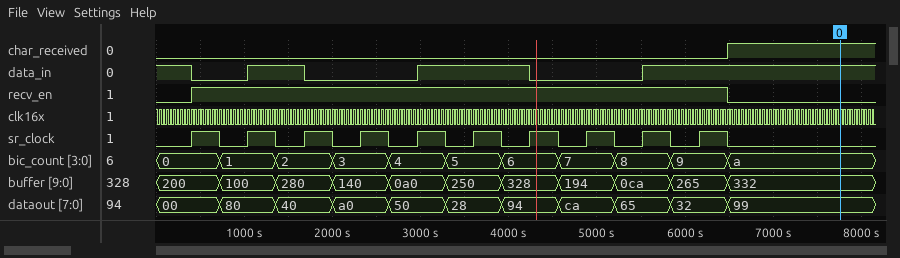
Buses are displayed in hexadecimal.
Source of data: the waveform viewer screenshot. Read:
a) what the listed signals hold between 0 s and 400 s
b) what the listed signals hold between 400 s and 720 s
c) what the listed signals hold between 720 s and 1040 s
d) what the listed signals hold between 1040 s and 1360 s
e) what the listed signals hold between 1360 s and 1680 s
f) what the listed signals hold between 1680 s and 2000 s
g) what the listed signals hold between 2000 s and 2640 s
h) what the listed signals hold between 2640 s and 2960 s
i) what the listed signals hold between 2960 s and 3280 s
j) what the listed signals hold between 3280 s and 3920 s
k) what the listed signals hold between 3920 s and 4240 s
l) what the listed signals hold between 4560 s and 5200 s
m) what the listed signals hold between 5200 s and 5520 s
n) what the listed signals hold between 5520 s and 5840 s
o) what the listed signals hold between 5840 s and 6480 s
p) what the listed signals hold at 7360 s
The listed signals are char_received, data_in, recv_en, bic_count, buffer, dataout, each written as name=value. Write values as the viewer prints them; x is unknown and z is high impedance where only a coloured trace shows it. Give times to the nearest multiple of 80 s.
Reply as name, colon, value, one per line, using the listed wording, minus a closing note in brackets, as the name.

what the listed signals hold between 0 s and 400 s: char_received=0, data_in=1, recv_en=0, bic_count=0, buffer=200, dataout=00
what the listed signals hold between 400 s and 720 s: char_received=0, data_in=0, recv_en=1, bic_count=0, buffer=200, dataout=00
what the listed signals hold between 720 s and 1040 s: char_received=0, data_in=0, recv_en=1, bic_count=1, buffer=100, dataout=80
what the listed signals hold between 1040 s and 1360 s: char_received=0, data_in=1, recv_en=1, bic_count=1, buffer=100, dataout=80
what the listed signals hold between 1360 s and 1680 s: char_received=0, data_in=1, recv_en=1, bic_count=2, buffer=280, dataout=40
what the listed signals hold between 1680 s and 2000 s: char_received=0, data_in=0, recv_en=1, bic_count=2, buffer=280, dataout=40
what the listed signals hold between 2000 s and 2640 s: char_received=0, data_in=0, recv_en=1, bic_count=3, buffer=140, dataout=a0
what the listed signals hold between 2640 s and 2960 s: char_received=0, data_in=0, recv_en=1, bic_count=4, buffer=0a0, dataout=50
what the listed signals hold between 2960 s and 3280 s: char_received=0, data_in=1, recv_en=1, bic_count=4, buffer=0a0, dataout=50
what the listed signals hold between 3280 s and 3920 s: char_received=0, data_in=1, recv_en=1, bic_count=5, buffer=250, dataout=28
what the listed signals hold between 3920 s and 4240 s: char_received=0, data_in=1, recv_en=1, bic_count=6, buffer=328, dataout=94
what the listed signals hold between 4560 s and 5200 s: char_received=0, data_in=0, recv_en=1, bic_count=7, buffer=194, dataout=ca
what the listed signals hold between 5200 s and 5520 s: char_received=0, data_in=0, recv_en=1, bic_count=8, buffer=0ca, dataout=65
what the listed signals hold between 5520 s and 5840 s: char_received=0, data_in=1, recv_en=1, bic_count=8, buffer=0ca, dataout=65
what the listed signals hold between 5840 s and 6480 s: char_received=0, data_in=1, recv_en=1, bic_count=9, buffer=265, dataout=32
what the listed signals hold at 7360 s: char_received=1, data_in=1, recv_en=0, bic_count=a, buffer=332, dataout=99
